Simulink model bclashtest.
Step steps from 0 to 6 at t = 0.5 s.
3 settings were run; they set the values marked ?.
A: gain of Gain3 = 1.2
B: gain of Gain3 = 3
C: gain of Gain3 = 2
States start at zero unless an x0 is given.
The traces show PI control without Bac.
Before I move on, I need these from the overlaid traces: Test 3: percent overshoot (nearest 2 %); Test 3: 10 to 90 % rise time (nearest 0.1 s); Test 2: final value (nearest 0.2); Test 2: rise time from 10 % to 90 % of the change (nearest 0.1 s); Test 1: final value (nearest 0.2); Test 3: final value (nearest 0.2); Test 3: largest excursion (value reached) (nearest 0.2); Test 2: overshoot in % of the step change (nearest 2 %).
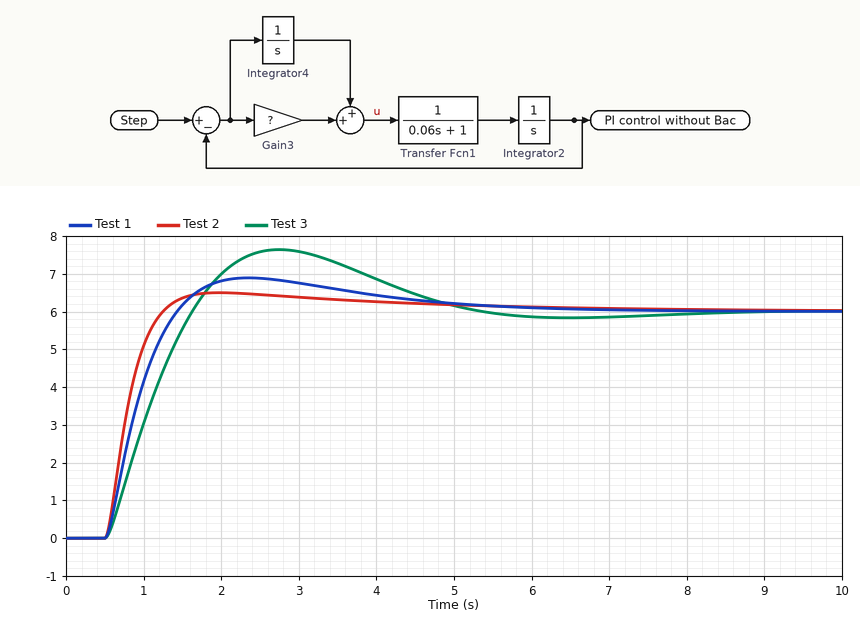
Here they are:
28 %
0.8 s
6.0
0.5 s
6.0
6.0
7.6
8 %
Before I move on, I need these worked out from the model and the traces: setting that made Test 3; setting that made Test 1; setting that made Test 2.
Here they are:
A
C
B
